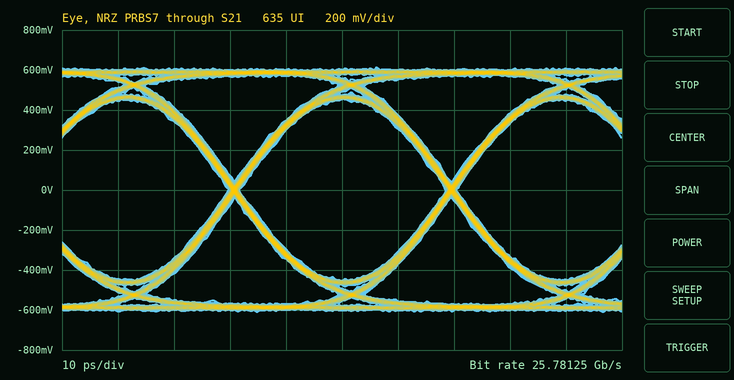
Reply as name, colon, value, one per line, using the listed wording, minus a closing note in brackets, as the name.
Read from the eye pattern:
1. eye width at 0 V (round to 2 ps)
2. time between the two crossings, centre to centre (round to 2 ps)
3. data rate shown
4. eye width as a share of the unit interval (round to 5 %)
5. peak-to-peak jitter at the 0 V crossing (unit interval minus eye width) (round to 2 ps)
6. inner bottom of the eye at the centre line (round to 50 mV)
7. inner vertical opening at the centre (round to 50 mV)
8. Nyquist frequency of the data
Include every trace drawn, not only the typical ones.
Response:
eye width at 0 V: 36 ps
time between the two crossings, centre to centre: 38 ps
data rate shown: 25.78125 Gb/s
eye width as a share of the unit interval: 95 %
peak-to-peak jitter at the 0 V crossing (unit interval minus eye width): 2 ps
inner bottom of the eye at the centre line: -450 mV
inner vertical opening at the centre: 900 mV
Nyquist frequency of the data: 12.89062 GHz
